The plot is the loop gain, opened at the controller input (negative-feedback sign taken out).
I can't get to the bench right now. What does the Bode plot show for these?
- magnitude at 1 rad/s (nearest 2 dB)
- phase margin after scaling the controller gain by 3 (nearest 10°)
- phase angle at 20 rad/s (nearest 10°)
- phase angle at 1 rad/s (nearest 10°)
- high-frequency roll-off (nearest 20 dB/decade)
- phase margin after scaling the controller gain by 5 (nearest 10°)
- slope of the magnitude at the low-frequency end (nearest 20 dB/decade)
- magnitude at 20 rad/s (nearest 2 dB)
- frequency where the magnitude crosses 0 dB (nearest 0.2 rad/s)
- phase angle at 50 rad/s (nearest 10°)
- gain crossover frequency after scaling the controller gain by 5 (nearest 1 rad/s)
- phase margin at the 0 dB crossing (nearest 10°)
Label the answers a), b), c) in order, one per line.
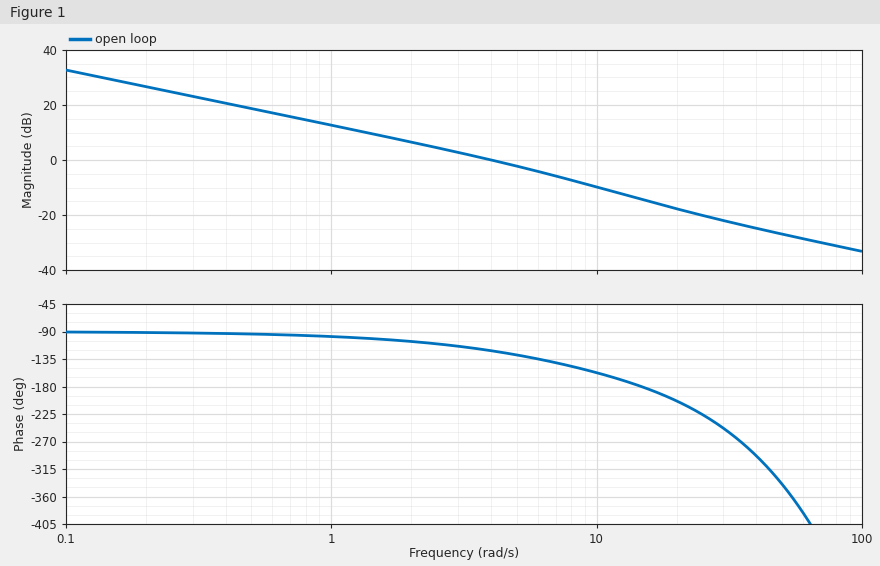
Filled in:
a) 12 dB
b) 20°
c) -200°
d) -100°
e) -20 dB/decade
f) 0°
g) -20 dB/decade
h) -18 dB
i) 4.0 rad/s
j) -340°
k) 14 rad/s
l) 60°
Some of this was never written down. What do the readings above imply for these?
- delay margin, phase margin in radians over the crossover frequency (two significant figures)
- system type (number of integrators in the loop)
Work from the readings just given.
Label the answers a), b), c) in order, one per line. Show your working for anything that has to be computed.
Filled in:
a) 60 × π / 180 / 4 = 0.26 s
b) 1
